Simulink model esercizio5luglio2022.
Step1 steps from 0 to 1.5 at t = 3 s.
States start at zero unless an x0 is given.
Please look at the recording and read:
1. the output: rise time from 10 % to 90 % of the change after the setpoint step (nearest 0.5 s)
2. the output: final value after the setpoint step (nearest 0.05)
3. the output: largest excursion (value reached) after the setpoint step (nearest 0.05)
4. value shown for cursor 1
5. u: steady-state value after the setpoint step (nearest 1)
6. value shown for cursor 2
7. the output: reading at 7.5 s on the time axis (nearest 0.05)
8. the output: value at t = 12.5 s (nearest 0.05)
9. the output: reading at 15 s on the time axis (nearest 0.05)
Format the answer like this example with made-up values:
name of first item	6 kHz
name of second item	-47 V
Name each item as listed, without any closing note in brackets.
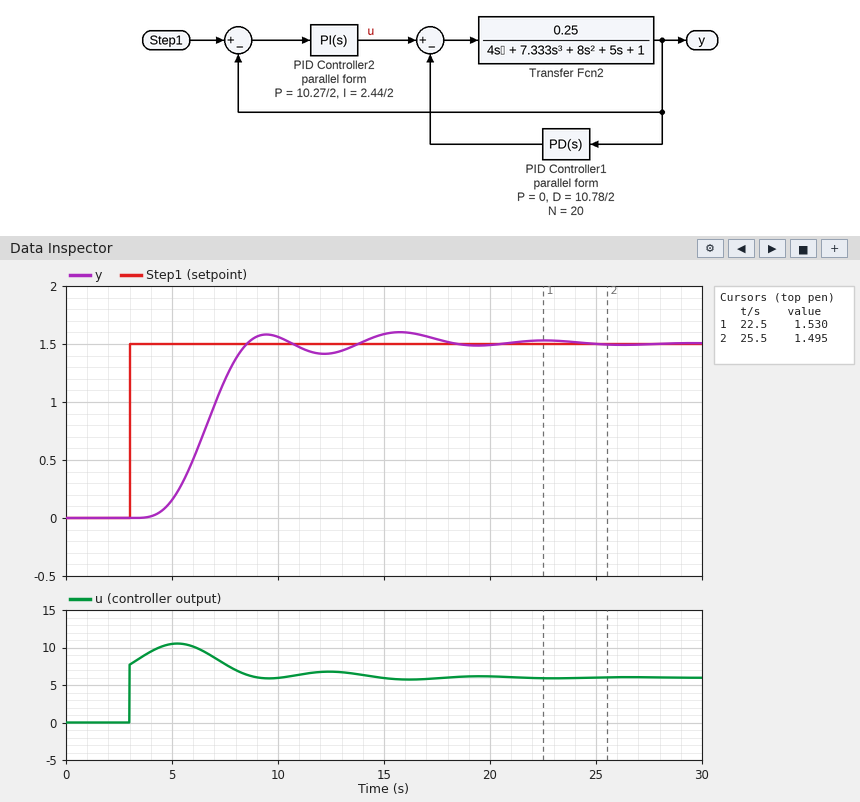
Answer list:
the output: rise time from 10 % to 90 % of the change after the setpoint step	3.0 s
the output: final value after the setpoint step	1.50
the output: largest excursion (value reached) after the setpoint step	1.60
value shown for cursor 1	1.530
u: steady-state value after the setpoint step	6
value shown for cursor 2	1.495
the output: reading at 7.5 s on the time axis	1.20
the output: value at t = 12.5 s	1.40
the output: reading at 15 s on the time axis	1.60
